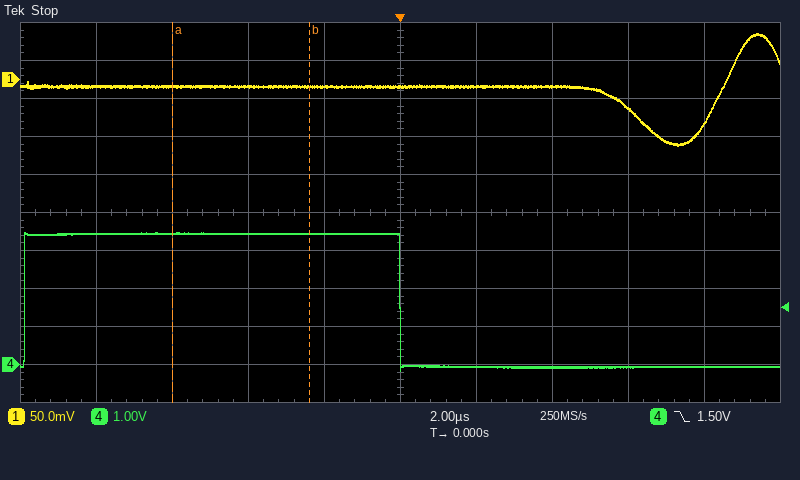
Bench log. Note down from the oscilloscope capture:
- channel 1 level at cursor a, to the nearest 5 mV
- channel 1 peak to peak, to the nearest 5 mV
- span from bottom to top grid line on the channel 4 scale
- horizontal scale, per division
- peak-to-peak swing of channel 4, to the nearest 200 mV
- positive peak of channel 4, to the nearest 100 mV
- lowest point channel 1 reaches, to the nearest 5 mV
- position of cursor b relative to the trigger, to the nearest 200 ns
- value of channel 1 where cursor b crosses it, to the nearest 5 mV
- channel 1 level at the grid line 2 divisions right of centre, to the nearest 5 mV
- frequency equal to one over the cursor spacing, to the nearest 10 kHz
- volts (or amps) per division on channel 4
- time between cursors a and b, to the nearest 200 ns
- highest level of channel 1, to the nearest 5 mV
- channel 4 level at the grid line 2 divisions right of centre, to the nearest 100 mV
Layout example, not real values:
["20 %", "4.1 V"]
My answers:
["-10 mV", "145 mV", "10 V", "2 µs", "3.6 V", "3.5 V", "-85 mV", "-2.4 µs", "-10 mV", "-10 mV", "280 kHz", "1 V", "3.6 µs", "60 mV", "-100 mV"]
